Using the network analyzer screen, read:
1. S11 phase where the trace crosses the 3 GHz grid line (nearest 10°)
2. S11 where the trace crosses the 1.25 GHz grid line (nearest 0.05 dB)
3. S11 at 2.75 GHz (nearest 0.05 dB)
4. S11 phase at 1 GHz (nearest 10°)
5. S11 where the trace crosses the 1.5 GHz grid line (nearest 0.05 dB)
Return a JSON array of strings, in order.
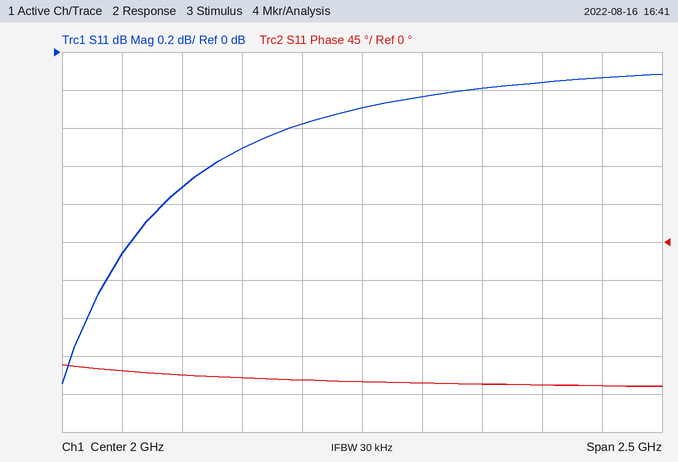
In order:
["-170°", "-0.70 dB", "-0.15 dB", "-150°", "-0.50 dB"]
